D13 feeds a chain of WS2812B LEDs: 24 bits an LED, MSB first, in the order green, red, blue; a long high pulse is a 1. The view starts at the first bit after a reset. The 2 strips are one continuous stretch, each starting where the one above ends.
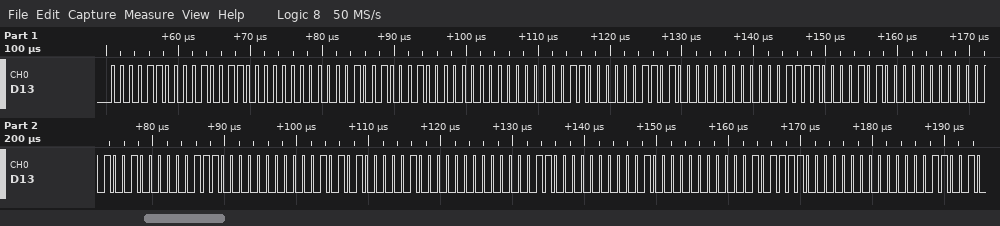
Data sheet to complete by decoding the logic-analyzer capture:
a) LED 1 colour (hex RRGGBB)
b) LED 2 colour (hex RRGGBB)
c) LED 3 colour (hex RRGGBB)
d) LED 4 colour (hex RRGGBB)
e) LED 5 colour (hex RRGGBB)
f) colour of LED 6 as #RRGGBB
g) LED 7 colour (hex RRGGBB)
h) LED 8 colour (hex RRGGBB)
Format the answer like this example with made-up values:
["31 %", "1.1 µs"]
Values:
["#260C00", "#201200", "#1A1800", "#141E00", "#0E2400", "#082A00", "#023000", "#002F03"]
